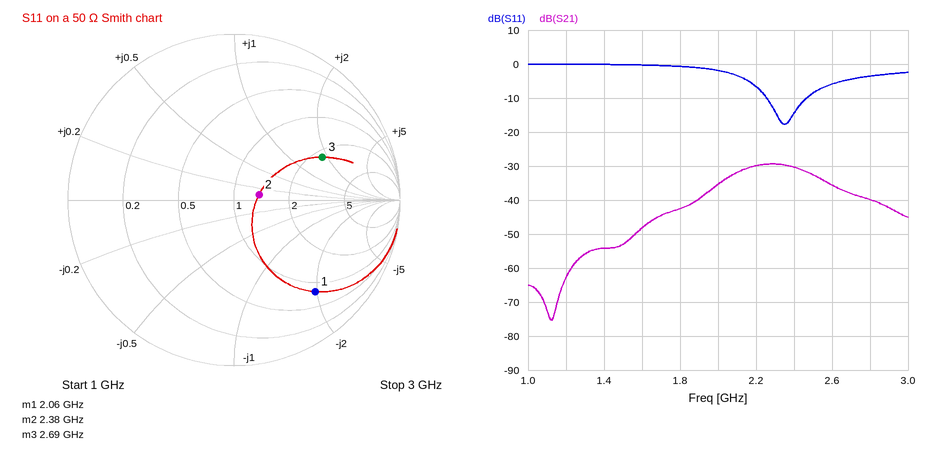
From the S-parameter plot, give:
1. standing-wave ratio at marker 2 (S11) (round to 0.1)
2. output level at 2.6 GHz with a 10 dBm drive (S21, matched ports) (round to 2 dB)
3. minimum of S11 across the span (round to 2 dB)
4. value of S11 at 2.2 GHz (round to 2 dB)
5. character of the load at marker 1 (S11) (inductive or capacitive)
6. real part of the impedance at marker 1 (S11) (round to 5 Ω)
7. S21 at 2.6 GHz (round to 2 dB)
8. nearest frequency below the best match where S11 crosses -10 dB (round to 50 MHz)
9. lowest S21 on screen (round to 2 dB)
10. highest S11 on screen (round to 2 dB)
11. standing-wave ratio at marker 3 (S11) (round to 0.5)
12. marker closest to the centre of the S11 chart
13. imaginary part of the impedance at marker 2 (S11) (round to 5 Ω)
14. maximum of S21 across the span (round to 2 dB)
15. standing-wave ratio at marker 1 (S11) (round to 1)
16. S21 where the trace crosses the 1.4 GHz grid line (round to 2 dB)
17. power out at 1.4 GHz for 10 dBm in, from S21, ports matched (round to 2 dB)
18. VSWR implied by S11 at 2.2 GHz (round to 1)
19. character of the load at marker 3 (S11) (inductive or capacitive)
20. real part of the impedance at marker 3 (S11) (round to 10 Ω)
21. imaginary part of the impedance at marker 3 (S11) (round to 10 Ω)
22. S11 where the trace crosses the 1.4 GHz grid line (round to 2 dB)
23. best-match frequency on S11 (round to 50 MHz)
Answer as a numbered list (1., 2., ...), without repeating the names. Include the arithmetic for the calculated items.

1. 1.4
2. 10 dBm + (-36 dB) = -26 dBm
3. -18 dB
4. -6 dB
5. capacitive
6. 40 Ω
7. -36 dB
8. 2.25 GHz
9. -76 dB
10. 0 dB
11. 4.0
12. marker 2
13. +5 Ω
14. -30 dB
15. 7
16. -54 dB
17. 10 dBm + (-54 dB) = -44 dBm
18. |Γ| = 10^(-6/20) = 0.5012; VSWR = (1 + 0.5012)/(1 − 0.5012) ≈ 3
19. inductive
20. 110 Ω
21. +90 Ω
22. 0 dB
23. 2.35 GHz
